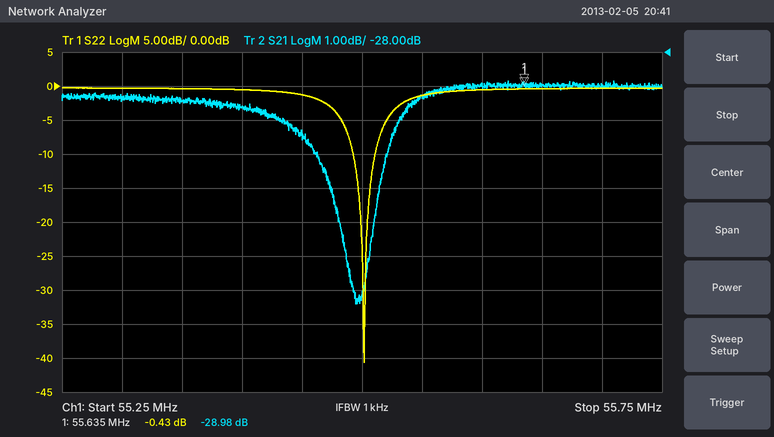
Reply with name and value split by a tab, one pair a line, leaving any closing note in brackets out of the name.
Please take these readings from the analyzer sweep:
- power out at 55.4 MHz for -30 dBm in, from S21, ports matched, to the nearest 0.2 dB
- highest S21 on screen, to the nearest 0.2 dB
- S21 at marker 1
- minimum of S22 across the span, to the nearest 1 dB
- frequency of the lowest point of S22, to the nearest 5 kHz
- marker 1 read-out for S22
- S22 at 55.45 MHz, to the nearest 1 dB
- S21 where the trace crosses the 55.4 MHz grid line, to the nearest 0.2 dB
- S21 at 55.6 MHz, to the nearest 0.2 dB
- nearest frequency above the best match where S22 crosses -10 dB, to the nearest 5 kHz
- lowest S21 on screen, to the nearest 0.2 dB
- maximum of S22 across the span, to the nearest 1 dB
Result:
power out at 55.4 MHz for -30 dBm in, from S21, ports matched, to the nearest 0.2 dB	-59.6 dBm
highest S21 on screen, to the nearest 0.2 dB	-28.8 dB
S21 at marker 1	-28.98 dB
minimum of S22 across the span, to the nearest 1 dB	-41 dB
frequency of the lowest point of S22, to the nearest 5 kHz	55.500 MHz
marker 1 read-out for S22	-0.43 dB
S22 at 55.45 MHz, to the nearest 1 dB	-1 dB
S21 where the trace crosses the 55.4 MHz grid line, to the nearest 0.2 dB	-29.6 dB
S21 at 55.6 MHz, to the nearest 0.2 dB	-29.0 dB
nearest frequency above the best match where S22 crosses -10 dB, to the nearest 5 kHz	55.510 MHz
lowest S21 on screen, to the nearest 0.2 dB	-35.4 dB
maximum of S22 across the span, to the nearest 1 dB	0 dB
